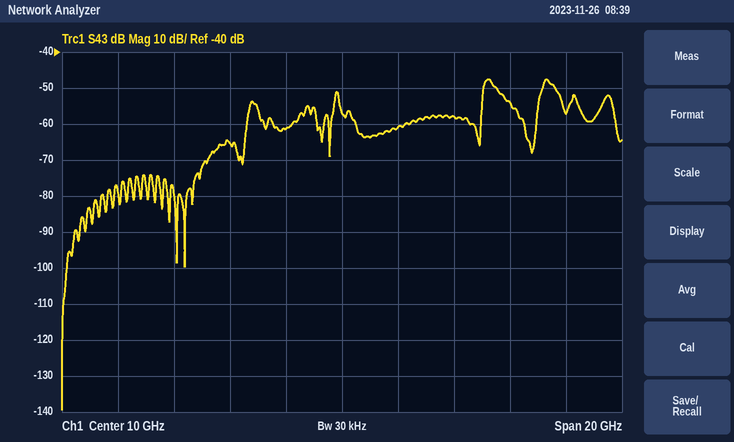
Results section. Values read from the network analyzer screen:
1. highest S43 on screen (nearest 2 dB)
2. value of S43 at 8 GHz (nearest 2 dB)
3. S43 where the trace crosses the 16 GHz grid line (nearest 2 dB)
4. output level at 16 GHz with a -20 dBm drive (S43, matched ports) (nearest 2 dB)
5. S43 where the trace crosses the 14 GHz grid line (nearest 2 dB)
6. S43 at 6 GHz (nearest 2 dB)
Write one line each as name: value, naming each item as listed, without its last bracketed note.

highest S43 on screen: -48 dB
value of S43 at 8 GHz: -62 dB
S43 where the trace crosses the 16 GHz grid line: -54 dB
output level at 16 GHz with a -20 dBm drive (S43, matched ports): -74 dBm
S43 where the trace crosses the 14 GHz grid line: -58 dB
S43 at 6 GHz: -66 dB
